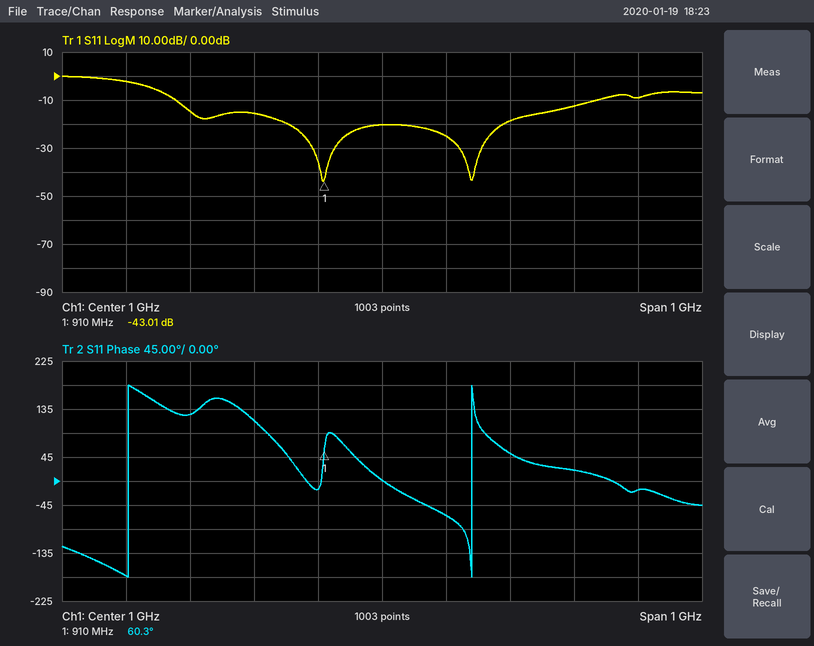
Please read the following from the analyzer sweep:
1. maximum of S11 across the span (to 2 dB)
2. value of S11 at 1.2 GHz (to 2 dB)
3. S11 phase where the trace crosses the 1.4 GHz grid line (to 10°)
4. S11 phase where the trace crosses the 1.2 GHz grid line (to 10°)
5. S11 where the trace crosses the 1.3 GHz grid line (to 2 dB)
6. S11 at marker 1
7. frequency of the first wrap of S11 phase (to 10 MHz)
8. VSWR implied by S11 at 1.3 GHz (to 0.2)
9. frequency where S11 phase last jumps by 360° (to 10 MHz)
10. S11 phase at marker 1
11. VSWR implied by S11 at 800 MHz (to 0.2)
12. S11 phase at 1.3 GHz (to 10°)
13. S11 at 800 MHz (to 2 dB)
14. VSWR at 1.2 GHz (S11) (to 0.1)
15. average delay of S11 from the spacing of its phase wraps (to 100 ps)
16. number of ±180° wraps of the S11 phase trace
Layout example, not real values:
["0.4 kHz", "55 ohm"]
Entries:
["0 dB", "-18 dB", "-20°", "50°", "-12 dB", "-43.01 dB", "600 MHz", "1.6", "1.14 GHz", "60.3°", "1.4", "20°", "-16 dB", "1.3", "1.9 ns", "2"]
